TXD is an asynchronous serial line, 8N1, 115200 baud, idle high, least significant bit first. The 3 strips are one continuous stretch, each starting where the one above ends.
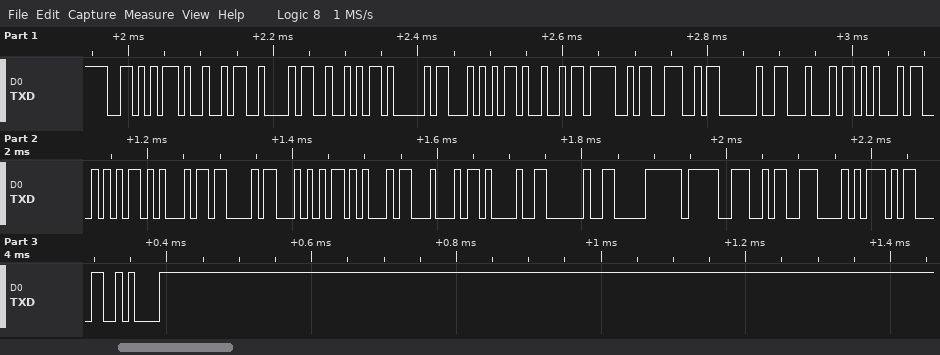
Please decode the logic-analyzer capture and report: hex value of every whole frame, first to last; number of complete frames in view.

56 49 42 52 41 54 49 4F 4E 20 44 45 54 45 43 54 45 44 21 20 F0 9F 9A A8 0D 0A
26
